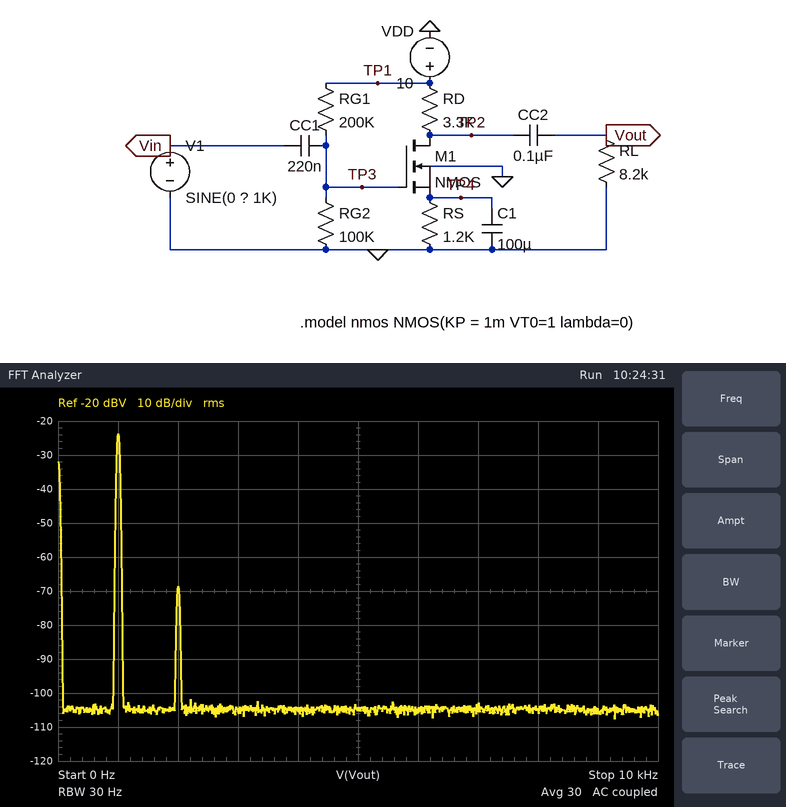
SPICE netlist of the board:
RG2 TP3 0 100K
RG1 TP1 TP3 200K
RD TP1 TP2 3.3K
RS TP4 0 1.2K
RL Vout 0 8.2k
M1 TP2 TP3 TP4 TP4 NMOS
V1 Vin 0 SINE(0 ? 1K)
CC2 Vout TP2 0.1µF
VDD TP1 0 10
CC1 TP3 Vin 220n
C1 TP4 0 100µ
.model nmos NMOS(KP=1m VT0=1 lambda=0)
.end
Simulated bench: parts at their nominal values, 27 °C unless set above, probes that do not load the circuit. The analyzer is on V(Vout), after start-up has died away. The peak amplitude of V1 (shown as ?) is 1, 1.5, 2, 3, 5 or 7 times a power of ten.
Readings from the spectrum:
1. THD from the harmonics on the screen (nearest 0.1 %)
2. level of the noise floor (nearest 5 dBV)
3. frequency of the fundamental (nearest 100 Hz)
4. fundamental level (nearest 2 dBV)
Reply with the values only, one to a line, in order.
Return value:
0.6 %
-105 dBV
1.0 kHz
-24 dBV
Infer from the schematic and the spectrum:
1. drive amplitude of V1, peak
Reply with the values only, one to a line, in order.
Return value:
30 mV
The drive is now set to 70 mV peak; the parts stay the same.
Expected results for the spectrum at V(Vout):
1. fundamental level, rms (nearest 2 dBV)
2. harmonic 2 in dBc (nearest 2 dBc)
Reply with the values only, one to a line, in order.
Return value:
-16 dBV
-38 dBc
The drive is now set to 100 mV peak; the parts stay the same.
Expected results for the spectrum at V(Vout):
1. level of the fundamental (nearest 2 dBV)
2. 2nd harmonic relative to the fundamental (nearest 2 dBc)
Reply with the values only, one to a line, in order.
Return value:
-14 dBV
-34 dBc
